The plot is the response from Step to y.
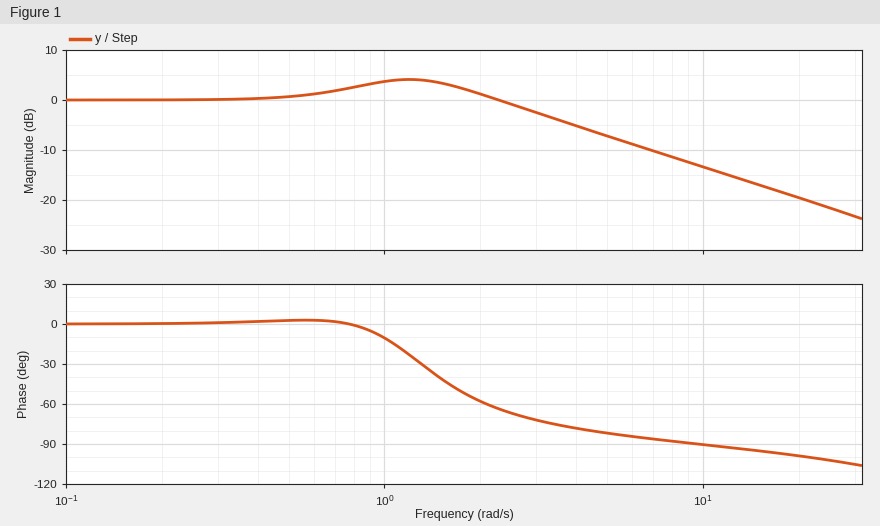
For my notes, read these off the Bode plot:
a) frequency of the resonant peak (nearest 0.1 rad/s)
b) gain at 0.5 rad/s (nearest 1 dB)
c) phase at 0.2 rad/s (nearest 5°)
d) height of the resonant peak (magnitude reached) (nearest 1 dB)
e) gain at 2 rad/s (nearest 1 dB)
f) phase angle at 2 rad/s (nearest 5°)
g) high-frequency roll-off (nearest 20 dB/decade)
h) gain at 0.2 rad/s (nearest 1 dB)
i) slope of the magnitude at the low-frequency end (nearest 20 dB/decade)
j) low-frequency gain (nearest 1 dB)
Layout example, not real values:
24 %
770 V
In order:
1.2 rad/s
1 dB
0°
4 dB
1 dB
-60°
-20 dB/decade
0 dB
0 dB/decade
0 dB
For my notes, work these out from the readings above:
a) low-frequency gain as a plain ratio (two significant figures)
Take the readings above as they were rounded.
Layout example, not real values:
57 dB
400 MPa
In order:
1.0
